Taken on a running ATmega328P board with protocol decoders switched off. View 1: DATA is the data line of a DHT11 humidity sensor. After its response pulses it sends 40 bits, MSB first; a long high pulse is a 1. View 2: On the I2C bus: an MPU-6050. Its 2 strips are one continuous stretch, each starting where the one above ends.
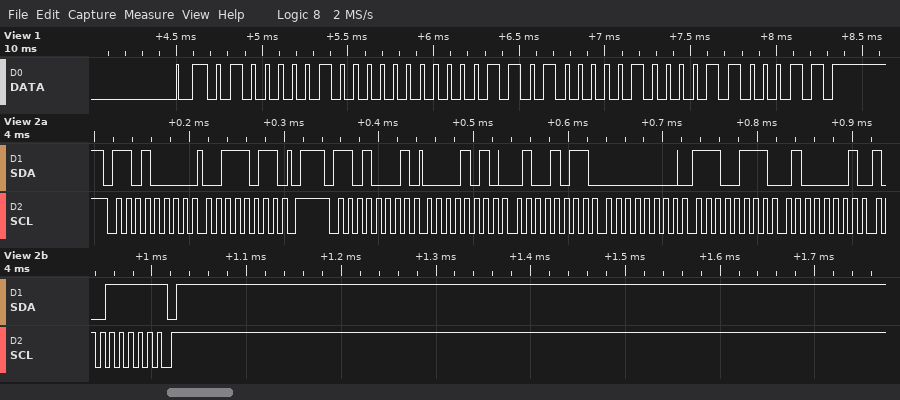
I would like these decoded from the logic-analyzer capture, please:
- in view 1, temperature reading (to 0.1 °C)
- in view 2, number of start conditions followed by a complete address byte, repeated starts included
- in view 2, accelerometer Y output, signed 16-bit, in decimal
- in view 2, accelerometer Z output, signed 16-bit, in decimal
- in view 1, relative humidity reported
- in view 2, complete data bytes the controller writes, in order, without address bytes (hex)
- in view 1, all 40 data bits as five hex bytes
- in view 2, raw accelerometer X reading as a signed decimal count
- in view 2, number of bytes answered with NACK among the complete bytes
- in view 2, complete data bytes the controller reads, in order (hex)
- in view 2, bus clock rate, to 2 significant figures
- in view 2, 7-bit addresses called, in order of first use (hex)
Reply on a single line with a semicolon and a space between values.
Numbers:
26.8 °C; 2; 231; 16799; 65 %; 3B; 41 00 1A 08 63; 2635; 1; 0A 4B 00 E7 41 9F; 100 kHz; 0x68
